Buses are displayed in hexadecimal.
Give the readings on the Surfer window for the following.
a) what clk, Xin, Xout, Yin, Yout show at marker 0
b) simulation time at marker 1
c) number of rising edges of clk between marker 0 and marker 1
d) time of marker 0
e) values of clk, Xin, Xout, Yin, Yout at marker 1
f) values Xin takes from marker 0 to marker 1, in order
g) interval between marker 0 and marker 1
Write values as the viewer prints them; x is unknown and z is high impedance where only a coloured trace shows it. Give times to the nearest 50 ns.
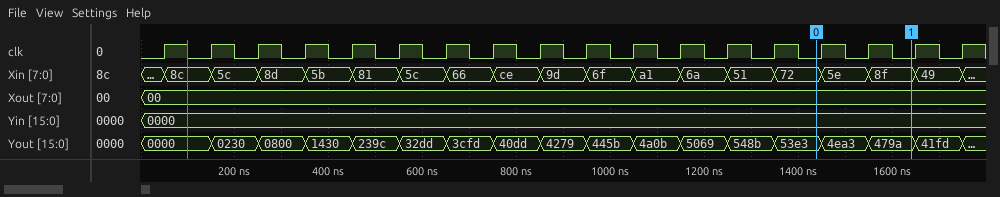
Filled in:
clk=0, Xin=72, Xout=00, Yin=0000, Yout=53e3
1650 ns
2
1450 ns
clk=0, Xin=8f, Xout=00, Yin=0000, Yout=479a
72, 5e, 8f
200 ns
